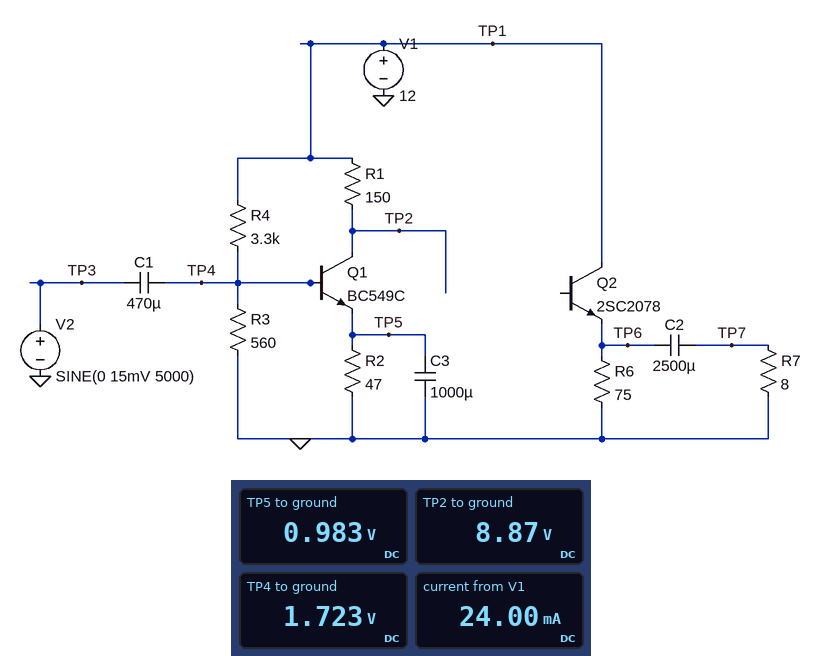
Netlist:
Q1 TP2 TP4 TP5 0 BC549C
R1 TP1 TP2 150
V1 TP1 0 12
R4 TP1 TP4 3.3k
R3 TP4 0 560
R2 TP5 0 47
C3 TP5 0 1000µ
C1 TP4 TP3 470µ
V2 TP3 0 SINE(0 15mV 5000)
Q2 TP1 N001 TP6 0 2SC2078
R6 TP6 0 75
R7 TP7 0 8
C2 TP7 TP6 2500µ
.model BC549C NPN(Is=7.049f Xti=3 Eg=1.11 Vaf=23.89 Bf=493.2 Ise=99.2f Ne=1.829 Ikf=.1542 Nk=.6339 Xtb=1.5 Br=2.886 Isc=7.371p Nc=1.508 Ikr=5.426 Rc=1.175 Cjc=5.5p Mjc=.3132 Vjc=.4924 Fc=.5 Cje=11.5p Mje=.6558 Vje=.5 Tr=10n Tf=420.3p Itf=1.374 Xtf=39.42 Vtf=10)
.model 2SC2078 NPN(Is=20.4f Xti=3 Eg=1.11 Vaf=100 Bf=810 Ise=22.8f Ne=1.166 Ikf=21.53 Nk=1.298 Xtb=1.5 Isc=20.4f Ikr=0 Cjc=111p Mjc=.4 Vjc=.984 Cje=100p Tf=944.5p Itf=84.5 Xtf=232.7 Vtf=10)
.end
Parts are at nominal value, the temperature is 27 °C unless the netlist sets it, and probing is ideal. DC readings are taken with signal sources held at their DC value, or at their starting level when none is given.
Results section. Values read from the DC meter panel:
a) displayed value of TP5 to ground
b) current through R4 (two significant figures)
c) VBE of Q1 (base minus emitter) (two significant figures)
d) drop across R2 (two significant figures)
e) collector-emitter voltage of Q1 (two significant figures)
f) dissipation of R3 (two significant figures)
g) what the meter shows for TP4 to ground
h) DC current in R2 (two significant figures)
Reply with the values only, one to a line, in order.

0.983 V
3.1 mA
740 mV
980 mV
7.9 V
5.3 mW
1.723 V
21 mA
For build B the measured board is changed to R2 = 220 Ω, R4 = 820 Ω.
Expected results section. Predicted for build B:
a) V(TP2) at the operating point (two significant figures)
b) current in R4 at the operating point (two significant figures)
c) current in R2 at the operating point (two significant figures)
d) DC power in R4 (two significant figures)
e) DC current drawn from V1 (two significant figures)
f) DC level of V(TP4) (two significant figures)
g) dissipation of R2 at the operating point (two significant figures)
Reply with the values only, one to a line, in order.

9.2 V
8.7 mA
19 mA
62 mW
27 mA
4.9 V
77 mW
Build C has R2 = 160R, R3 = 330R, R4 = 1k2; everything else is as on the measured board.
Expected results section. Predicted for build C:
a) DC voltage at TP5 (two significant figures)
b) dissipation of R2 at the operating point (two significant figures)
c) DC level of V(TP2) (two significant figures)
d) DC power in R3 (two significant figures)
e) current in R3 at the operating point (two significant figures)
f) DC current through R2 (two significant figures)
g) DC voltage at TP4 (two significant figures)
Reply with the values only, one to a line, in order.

1.9 V
22 mW
10 V
20 mW
7.8 mA
12 mA
2.6 V
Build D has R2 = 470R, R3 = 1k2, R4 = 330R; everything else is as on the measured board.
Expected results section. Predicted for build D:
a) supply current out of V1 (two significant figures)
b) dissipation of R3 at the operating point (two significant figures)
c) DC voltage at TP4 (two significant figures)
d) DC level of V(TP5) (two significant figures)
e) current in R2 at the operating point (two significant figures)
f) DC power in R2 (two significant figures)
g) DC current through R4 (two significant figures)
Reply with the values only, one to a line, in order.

26 mA
74 mW
9.4 V
8.7 V
18 mA
160 mW
7.9 mA
